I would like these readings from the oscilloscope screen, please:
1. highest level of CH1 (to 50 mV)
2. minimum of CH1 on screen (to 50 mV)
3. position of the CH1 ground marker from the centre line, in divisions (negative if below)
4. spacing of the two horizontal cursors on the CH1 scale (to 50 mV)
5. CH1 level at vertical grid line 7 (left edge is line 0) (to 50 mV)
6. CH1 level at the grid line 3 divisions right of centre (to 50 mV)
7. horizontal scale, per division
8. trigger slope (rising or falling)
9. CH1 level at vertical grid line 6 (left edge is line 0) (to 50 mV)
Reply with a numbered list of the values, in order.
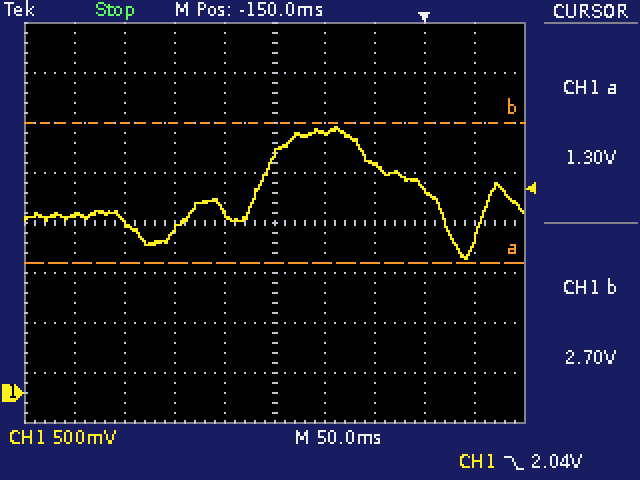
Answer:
1. 2.65 V
2. 1.35 V
3. -3.4 div
4. 1.40 V
5. 2.30 V
6. 2.05 V
7. 50 ms
8. falling
9. 2.60 V
